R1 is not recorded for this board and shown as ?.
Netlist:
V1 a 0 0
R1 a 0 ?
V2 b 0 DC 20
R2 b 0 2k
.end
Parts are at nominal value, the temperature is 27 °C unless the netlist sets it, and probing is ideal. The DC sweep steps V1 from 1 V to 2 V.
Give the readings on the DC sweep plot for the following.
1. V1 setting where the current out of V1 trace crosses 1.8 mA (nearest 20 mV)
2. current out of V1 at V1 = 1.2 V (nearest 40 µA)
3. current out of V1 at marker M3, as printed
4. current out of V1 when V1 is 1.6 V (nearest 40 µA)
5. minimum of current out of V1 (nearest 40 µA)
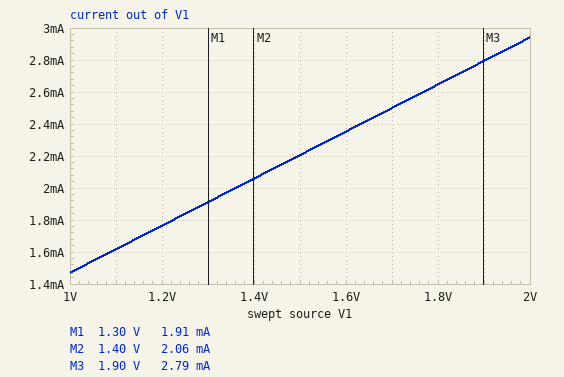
1.22 V
1.76 mA
2.79 mA
2.36 mA
1.48 mA
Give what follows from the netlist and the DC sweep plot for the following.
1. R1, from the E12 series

680 Ω
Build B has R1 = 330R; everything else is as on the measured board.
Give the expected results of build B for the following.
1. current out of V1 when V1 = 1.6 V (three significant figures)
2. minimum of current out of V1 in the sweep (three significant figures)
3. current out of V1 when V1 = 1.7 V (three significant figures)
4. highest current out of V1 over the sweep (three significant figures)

4.85 mA
3.03 mA
5.15 mA
6.06 mA
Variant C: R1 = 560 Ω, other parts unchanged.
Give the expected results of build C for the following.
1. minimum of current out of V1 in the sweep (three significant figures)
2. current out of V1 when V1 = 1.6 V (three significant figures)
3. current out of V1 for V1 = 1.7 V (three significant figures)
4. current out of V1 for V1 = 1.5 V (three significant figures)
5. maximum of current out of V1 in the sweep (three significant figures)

1.79 mA
2.86 mA
3.04 mA
2.68 mA
3.57 mA
